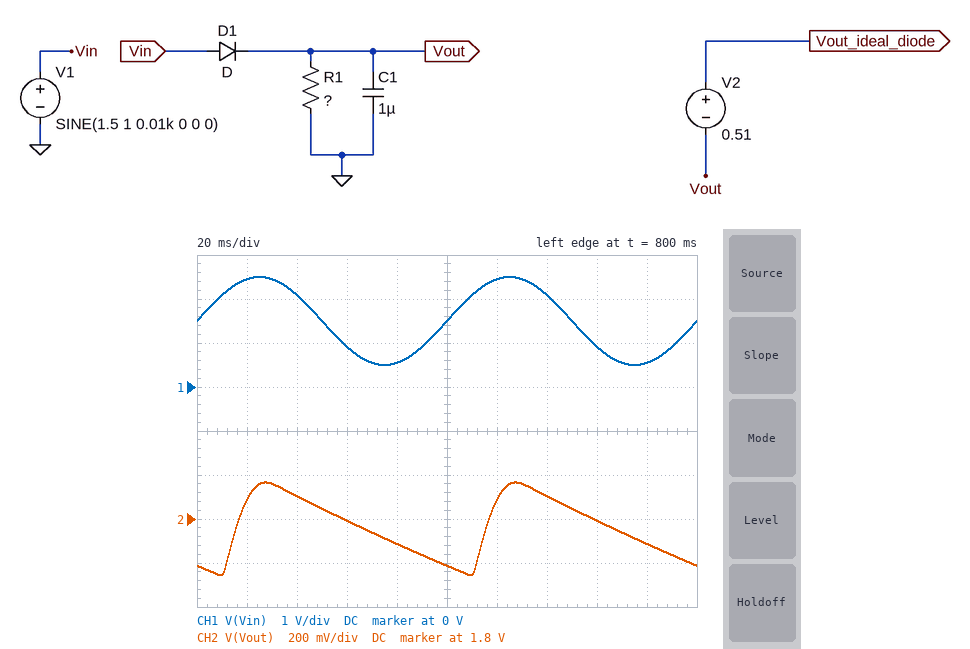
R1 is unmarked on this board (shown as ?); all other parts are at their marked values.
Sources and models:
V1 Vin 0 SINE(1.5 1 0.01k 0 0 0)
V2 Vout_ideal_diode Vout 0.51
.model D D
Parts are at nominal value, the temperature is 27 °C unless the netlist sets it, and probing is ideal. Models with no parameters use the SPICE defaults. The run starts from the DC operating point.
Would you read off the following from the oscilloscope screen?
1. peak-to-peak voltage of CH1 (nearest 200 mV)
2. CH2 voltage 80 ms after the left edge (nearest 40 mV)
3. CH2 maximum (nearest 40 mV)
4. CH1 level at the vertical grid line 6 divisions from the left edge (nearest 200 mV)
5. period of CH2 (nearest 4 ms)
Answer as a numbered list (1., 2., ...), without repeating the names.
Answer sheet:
1. 2.0 V
2. 1.68 V
3. 1.96 V
4. 2.4 V
5. 100 ms
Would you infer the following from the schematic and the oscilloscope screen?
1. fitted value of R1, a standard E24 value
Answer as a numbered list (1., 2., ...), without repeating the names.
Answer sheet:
1. 330 kΩ
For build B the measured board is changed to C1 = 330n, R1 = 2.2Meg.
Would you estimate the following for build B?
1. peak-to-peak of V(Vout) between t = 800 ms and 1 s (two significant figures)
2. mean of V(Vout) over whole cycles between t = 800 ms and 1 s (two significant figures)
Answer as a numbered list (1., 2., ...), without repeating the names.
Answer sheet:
1. 220 mV
2. 1.9 V
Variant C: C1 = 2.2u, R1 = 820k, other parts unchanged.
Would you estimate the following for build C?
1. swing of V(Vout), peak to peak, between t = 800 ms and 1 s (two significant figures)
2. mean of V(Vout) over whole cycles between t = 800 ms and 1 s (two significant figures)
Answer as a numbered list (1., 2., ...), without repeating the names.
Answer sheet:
1. 91 mV
2. 1.9 V
